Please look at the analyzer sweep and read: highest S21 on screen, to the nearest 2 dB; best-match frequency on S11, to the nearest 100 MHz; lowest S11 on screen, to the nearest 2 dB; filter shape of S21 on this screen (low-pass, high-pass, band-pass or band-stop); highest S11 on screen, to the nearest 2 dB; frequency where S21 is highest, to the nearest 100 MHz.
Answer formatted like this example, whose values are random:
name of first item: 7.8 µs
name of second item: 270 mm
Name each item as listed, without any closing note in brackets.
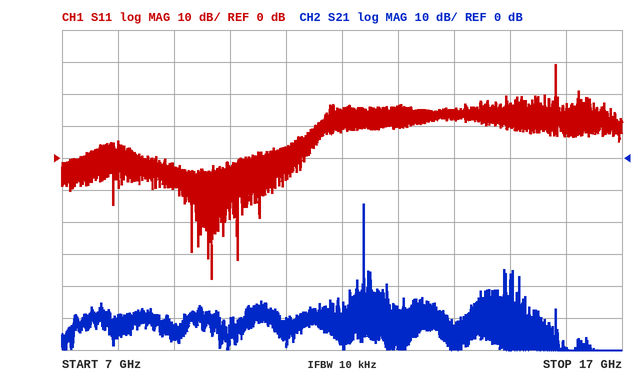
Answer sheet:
highest S21 on screen, to the nearest 2 dB: -14 dB
best-match frequency on S11, to the nearest 100 MHz: 9.7 GHz
lowest S11 on screen, to the nearest 2 dB: -38 dB
filter shape of S21 on this screen: band-pass
highest S11 on screen, to the nearest 2 dB: 30 dB
frequency where S21 is highest, to the nearest 100 MHz: 12.4 GHz
